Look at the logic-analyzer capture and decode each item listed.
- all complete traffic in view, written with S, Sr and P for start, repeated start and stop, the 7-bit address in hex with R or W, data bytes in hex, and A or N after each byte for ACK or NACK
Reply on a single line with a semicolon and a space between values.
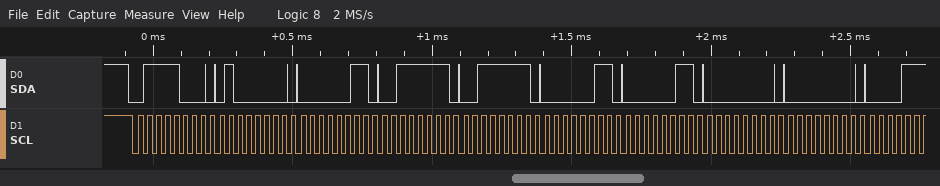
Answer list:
S 3CW A 40 A 03 A 3F A 3F A 03 A 03 A 00 A 00 A
